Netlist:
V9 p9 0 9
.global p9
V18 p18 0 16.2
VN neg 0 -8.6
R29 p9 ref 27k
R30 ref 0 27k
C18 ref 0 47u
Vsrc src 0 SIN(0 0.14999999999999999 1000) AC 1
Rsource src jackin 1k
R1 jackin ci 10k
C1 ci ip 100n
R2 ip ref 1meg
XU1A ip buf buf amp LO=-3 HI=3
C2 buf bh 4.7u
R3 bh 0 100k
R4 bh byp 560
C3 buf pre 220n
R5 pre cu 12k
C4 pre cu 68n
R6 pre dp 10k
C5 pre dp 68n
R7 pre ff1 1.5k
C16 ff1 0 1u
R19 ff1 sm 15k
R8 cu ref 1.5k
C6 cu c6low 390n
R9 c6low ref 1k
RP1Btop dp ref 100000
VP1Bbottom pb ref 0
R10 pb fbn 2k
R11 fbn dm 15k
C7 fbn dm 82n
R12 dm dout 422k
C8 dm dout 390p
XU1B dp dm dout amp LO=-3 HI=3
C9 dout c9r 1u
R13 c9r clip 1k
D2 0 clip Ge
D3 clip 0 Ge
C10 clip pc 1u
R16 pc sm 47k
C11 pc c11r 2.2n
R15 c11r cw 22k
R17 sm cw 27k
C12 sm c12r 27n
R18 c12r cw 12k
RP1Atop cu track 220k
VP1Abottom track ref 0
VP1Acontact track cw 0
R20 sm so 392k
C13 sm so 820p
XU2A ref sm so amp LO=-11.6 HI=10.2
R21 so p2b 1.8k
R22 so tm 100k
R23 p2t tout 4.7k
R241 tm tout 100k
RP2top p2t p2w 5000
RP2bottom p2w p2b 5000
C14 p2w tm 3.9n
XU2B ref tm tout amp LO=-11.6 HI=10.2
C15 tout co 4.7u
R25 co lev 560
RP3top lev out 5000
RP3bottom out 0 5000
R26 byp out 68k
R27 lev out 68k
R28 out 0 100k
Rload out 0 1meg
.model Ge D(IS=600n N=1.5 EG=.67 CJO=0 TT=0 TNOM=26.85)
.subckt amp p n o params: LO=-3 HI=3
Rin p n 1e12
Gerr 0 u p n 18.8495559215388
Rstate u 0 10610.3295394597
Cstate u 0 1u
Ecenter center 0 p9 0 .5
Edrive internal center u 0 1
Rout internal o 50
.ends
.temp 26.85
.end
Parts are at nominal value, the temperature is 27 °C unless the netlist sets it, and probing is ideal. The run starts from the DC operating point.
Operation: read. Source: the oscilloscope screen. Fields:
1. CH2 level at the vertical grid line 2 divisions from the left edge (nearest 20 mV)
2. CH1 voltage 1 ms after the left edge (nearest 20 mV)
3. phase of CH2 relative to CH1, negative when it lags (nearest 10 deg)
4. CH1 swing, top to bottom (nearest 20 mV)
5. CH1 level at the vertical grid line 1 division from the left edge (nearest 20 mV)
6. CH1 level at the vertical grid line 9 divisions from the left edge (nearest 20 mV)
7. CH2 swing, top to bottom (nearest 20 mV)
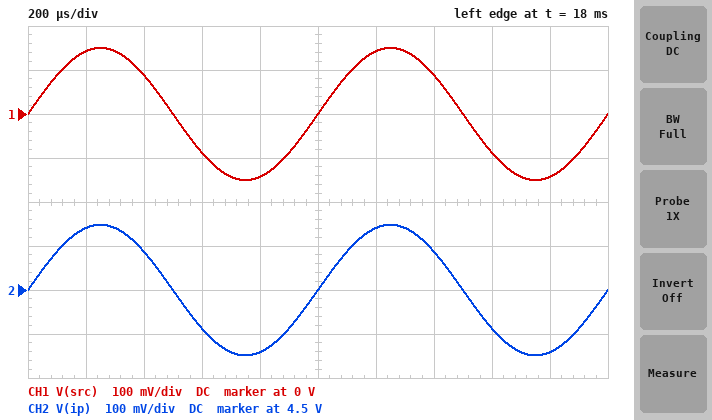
4.58 V
0 V
0 deg
300 mV
140 mV
-140 mV
300 mV
